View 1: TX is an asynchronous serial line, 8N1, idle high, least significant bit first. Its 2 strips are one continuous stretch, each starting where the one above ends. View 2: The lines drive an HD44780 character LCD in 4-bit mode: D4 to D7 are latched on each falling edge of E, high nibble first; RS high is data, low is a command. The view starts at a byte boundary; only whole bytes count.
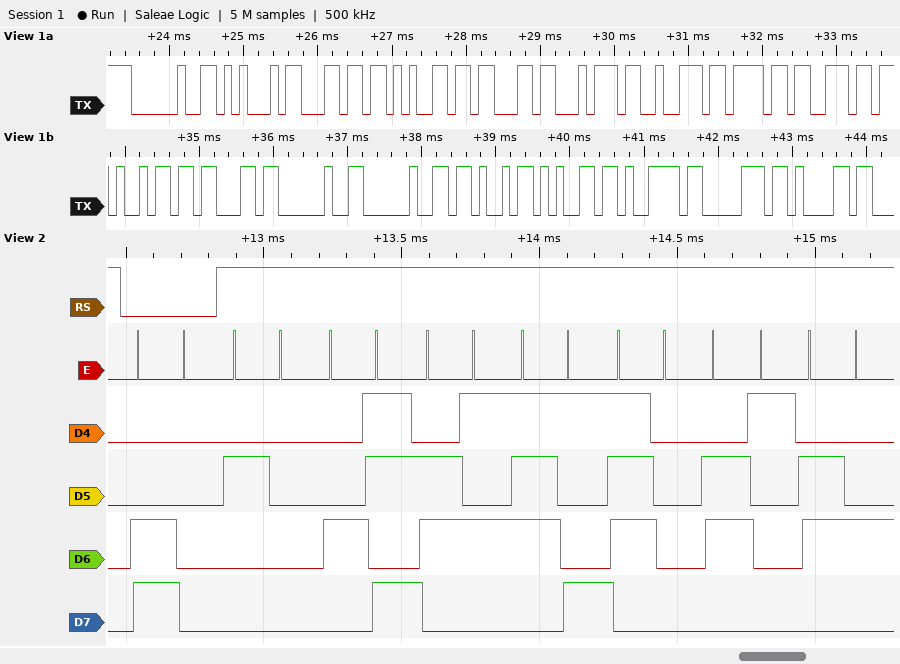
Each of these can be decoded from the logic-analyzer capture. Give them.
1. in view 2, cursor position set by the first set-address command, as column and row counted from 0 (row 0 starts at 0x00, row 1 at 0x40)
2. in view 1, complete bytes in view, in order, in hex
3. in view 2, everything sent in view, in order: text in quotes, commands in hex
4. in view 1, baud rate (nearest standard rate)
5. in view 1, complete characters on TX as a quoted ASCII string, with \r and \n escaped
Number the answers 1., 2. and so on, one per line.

1. column 0, row 1
2. 20 45 6C 65 63 74 72 6F 6E 69 63 20 20 4B 65 79 70 61
3. 0xC0 " Keypad"
4. 9600 baud
5. " Electronic  Keypa"
